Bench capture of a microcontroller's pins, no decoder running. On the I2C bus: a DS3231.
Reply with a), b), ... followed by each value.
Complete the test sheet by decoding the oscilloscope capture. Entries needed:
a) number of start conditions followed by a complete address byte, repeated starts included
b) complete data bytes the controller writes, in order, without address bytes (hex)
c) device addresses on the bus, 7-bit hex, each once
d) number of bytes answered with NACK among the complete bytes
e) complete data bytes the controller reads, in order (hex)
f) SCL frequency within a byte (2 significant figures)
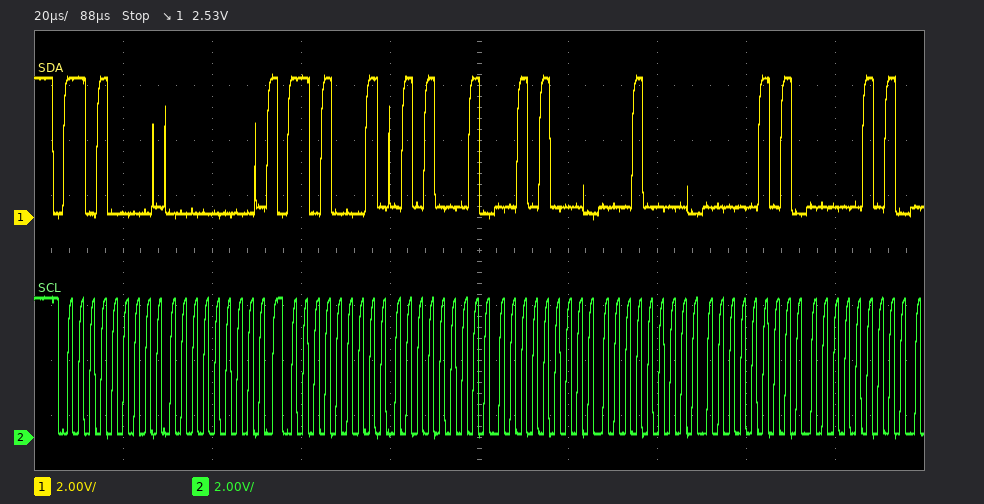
a) 2
b) 00
c) 0x68
d) 0
e) 51 28 10 05 05
f) 400 kHz
